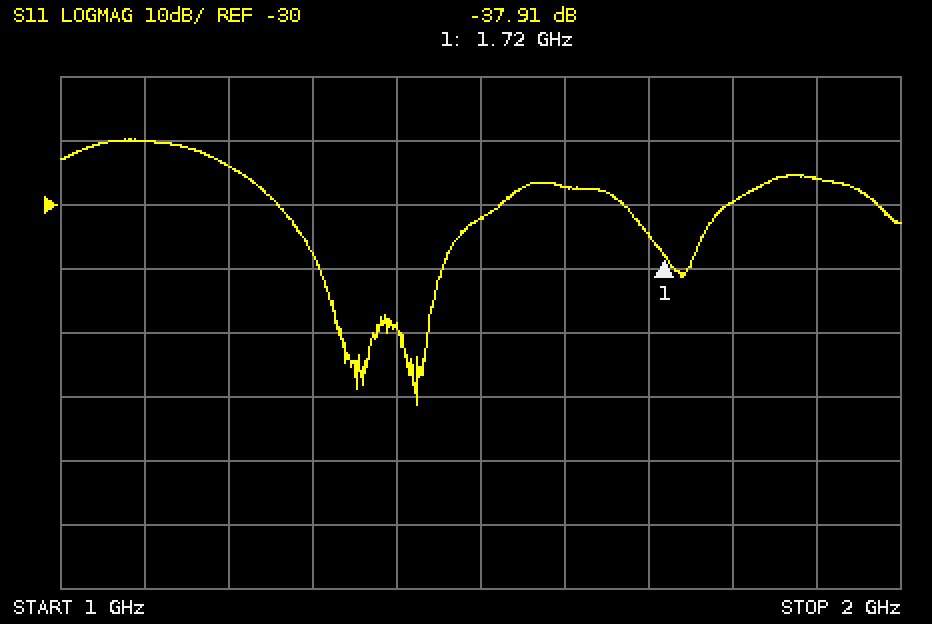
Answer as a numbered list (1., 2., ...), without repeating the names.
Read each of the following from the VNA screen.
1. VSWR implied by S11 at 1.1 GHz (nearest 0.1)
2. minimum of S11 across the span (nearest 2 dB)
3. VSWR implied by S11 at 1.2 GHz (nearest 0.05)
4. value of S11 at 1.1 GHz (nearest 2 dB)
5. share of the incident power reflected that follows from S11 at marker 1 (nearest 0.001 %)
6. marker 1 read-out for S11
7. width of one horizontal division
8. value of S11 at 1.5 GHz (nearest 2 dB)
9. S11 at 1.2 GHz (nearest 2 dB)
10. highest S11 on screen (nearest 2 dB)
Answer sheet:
1. 1.2
2. -62 dB
3. 1.15
4. -20 dB
5. 0.016 %
6. -37.91 dB
7. 100 MHz
8. -32 dB
9. -24 dB
10. -20 dB
